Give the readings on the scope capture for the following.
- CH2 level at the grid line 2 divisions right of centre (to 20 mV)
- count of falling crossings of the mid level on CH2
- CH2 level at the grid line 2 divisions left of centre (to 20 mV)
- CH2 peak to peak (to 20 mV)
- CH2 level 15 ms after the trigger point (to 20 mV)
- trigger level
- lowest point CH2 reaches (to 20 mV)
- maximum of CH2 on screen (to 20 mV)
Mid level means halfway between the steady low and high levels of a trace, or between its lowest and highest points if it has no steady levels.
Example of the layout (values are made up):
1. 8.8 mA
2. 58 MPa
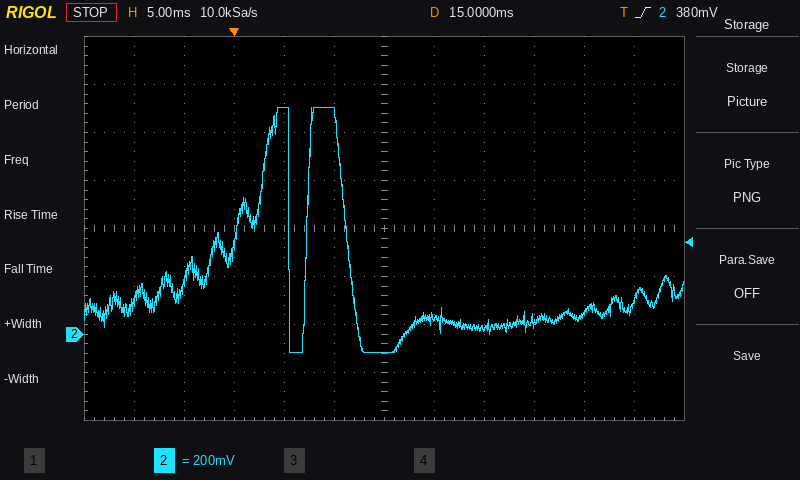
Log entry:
1. 20 mV
2. 2
3. 940 mV
4. 1.02 V
5. -80 mV
6. 380 mV
7. -80 mV
8. 940 mV
